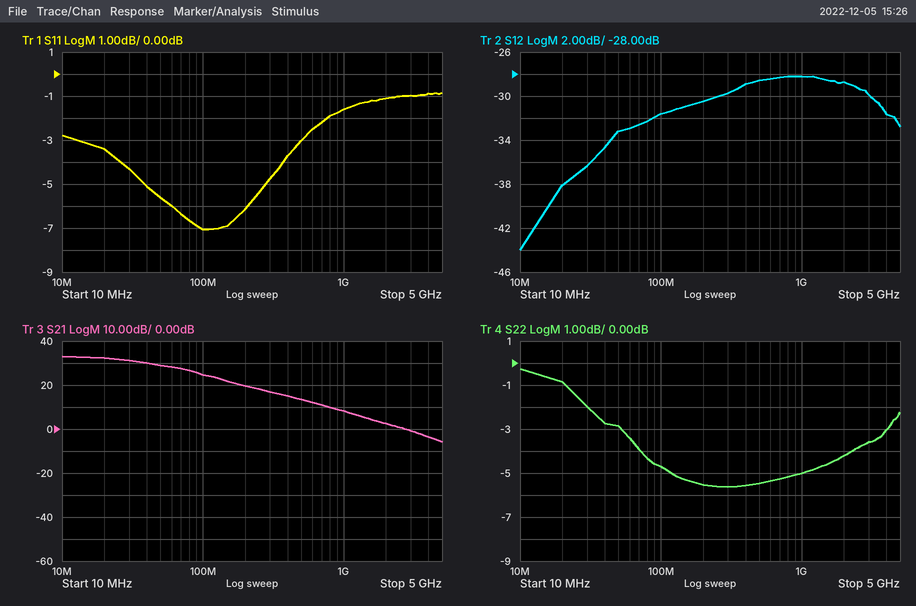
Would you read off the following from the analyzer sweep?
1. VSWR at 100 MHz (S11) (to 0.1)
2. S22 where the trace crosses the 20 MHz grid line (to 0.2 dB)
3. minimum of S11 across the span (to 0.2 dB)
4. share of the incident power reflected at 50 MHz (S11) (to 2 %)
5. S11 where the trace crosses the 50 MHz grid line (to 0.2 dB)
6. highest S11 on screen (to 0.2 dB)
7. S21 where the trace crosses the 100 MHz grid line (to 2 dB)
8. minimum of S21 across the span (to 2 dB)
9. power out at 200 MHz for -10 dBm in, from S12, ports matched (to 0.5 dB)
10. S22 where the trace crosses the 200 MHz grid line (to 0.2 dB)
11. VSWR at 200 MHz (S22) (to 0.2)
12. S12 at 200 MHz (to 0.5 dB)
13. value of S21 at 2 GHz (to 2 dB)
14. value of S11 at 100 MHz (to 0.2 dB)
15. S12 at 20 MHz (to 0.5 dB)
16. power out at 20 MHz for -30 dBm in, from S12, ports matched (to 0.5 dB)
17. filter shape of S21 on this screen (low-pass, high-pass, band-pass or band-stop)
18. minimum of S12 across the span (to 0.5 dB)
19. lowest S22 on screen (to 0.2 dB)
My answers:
2.6
-0.8 dB
-7.0 dB
28 %
-5.6 dB
-0.8 dB
24 dB
-6 dB
-40.5 dBm
-5.6 dB
3.2
-30.5 dB
2 dB
-7.0 dB
-38.0 dB
-68.0 dBm
low-pass
-44.0 dB
-5.6 dB
